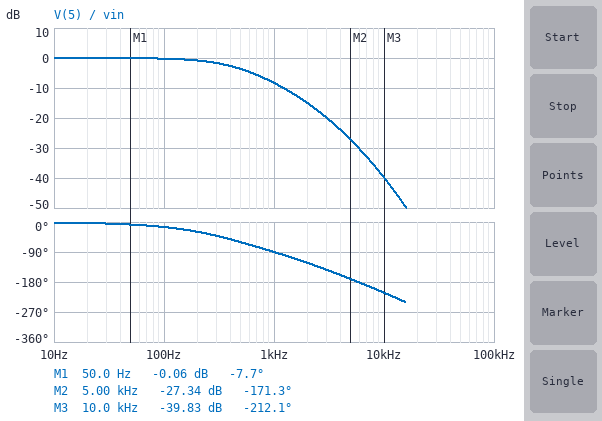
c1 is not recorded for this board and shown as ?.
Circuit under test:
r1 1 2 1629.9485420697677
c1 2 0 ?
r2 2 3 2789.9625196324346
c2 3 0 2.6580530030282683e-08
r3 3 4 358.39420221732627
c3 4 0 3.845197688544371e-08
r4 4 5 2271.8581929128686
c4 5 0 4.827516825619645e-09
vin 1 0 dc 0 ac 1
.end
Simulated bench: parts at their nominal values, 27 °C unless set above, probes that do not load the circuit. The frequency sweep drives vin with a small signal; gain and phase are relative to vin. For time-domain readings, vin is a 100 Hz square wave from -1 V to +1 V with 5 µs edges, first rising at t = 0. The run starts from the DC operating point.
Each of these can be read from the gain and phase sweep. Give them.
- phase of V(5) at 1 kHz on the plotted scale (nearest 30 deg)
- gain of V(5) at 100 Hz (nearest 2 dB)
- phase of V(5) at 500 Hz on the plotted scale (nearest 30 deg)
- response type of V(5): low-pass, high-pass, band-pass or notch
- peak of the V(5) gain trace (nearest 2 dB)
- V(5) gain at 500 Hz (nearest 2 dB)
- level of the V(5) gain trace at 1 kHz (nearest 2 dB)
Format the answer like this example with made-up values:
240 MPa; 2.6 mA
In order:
-90 deg; 0 dB; -60 deg; low-pass; 0 dB; -4 dB; -8 dB
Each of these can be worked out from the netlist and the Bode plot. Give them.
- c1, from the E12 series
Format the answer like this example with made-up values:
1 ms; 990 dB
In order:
56 nF
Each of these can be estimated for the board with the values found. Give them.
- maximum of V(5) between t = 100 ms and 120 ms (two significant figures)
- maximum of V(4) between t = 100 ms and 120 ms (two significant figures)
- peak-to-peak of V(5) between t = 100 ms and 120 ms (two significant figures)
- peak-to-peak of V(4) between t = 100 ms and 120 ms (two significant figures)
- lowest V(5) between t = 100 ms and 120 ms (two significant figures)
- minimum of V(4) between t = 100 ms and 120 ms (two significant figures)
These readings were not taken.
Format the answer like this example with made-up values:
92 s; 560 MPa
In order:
1.0 V; 1.0 V; 2.0 V; 2.0 V; -1.0 V; -1.0 V
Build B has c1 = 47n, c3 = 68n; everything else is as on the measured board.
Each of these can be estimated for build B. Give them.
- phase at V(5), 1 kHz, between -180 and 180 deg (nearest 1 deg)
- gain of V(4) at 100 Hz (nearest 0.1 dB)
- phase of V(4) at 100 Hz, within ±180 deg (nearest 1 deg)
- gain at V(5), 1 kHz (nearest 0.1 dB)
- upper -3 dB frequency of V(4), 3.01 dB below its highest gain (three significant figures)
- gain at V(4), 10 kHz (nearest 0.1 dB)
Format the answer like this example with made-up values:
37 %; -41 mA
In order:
-94 deg; -0.4 dB; -19 deg; -10.6 dB; 322 Hz; -40.1 dB
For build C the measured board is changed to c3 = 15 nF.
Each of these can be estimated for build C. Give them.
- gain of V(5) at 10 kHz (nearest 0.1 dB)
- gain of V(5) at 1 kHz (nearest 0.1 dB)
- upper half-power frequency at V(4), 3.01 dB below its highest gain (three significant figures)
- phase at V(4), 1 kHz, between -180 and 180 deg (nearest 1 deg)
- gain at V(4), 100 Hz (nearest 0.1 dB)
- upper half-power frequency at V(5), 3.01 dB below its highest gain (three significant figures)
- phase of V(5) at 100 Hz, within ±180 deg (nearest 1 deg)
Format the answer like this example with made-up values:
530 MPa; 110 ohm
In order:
-35.9 dB; -5.9 dB; 609 Hz; -76 deg; -0.1 dB; 608 Hz; -11 deg
